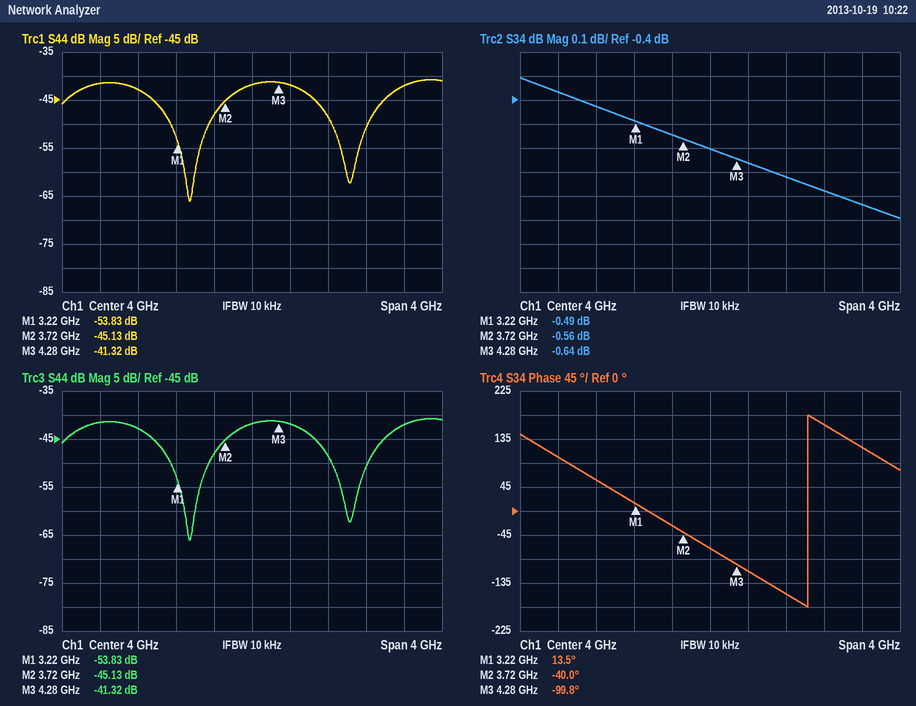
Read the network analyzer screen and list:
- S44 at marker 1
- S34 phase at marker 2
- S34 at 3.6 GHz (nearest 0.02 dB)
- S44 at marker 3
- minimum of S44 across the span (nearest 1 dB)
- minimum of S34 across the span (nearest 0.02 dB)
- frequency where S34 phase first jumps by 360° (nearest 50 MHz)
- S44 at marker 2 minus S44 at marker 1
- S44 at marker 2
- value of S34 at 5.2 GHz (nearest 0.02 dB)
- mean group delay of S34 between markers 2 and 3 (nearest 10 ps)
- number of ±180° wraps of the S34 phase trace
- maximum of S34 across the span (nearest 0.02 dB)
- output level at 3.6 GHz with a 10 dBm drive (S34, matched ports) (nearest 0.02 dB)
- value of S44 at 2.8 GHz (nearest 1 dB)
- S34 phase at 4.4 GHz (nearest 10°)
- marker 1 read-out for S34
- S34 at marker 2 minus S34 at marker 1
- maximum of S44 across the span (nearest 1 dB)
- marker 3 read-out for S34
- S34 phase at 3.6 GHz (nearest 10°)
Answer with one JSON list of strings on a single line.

["-53.83 dB", "-40.0°", "-0.54 dB", "-41.32 dB", "-66 dB", "-0.90 dB", "5.05 GHz", "8.70 dB", "-45.13 dB", "-0.78 dB", "300 ps", "1", "-0.30 dB", "9.46 dBm", "-43 dB", "-110°", "-0.49 dB", "-0.07 dB", "-41 dB", "-0.64 dB", "-30°"]
